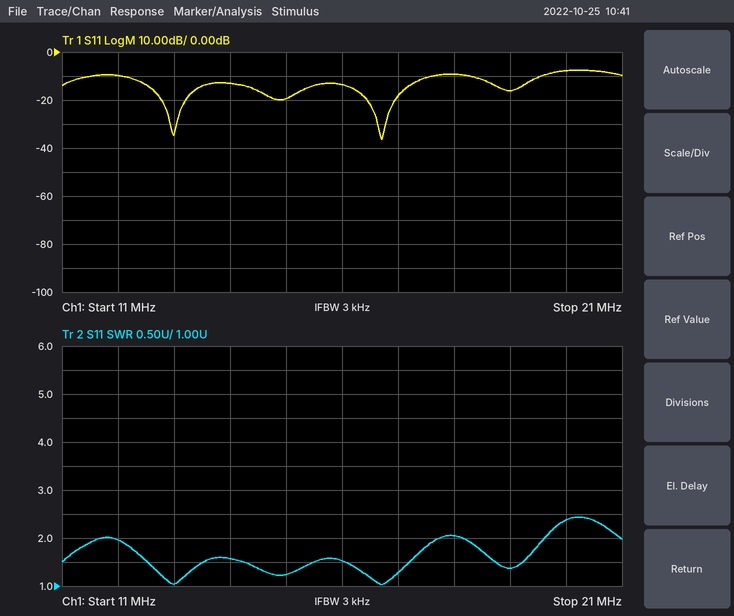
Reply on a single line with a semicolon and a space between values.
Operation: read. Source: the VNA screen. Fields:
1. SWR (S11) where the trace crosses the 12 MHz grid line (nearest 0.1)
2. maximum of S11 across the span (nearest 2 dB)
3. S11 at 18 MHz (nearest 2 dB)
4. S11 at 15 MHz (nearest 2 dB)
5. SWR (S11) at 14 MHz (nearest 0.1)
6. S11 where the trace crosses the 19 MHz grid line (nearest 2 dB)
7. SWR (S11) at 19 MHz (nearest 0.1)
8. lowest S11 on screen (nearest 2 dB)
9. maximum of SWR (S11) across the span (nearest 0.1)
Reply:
2.0; -8 dB; -10 dB; -20 dB; 1.6; -16 dB; 1.4; -36 dB; 2.4
